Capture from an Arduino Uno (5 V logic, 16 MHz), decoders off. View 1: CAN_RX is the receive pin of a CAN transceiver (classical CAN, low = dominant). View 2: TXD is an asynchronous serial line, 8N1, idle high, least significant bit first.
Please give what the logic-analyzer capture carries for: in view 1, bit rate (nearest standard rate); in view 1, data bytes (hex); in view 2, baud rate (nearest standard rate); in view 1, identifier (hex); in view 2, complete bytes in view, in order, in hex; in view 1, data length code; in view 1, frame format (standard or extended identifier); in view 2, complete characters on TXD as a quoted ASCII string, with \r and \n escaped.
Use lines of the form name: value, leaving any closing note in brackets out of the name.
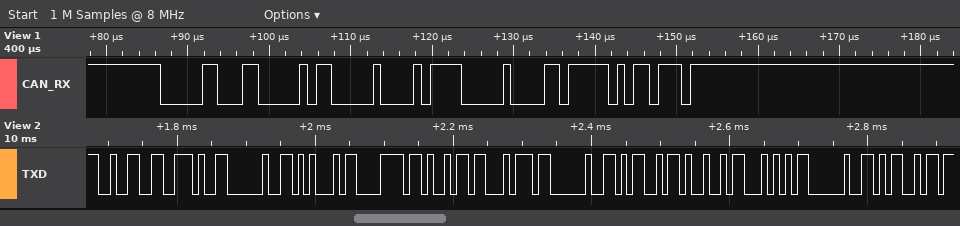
in view 1, bit rate: 1000 kbit/s
in view 1, data bytes: 00 5E 00
in view 2, baud rate: 115200 baud
in view 1, identifier: 0x046
in view 2, complete bytes in view, in order, in hex: 32 2E 20 45 78 69 74 20 4D 49 54 20 4D
in view 1, data length code: 3
in view 1, frame format: standard
in view 2, complete characters on TXD as a quoted ASCII string, with \r and \n escaped: "2. Exit MIT M"
